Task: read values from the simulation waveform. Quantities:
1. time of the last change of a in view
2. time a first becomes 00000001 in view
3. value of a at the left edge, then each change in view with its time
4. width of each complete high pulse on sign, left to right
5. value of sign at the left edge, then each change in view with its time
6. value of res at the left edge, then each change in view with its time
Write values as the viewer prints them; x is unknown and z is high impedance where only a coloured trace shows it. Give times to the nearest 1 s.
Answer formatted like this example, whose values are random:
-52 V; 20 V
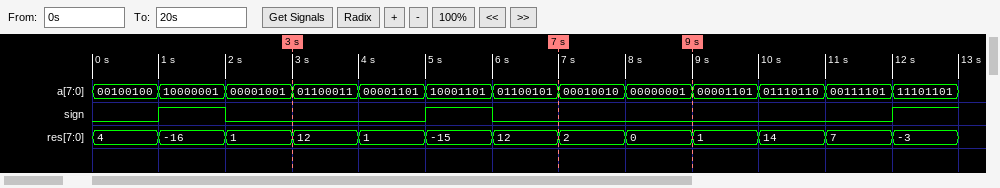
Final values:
12 s; 8 s; 00100100, 10000001 at 1 s, 00001001 at 2 s, 01100011 at 3 s, 00001101 at 4 s, 10001101 at 5 s, 01100101 at 6 s, 00010010 at 7 s, 00000001 at 8 s, 00001101 at 9 s, 01110110 at 10 s, 00111101 at 11 s, 11101101 at 12 s; 1 s, 1 s; 0, 1 at 1 s, 0 at 2 s, 1 at 5 s, 0 at 6 s, 1 at 12 s; 4, -16 at 1 s, 1 at 2 s, 12 at 3 s, 1 at 4 s, -15 at 5 s, 12 at 6 s, 2 at 7 s, 0 at 8 s, 1 at 9 s, 14 at 10 s, 7 at 11 s, -3 at 12 s
